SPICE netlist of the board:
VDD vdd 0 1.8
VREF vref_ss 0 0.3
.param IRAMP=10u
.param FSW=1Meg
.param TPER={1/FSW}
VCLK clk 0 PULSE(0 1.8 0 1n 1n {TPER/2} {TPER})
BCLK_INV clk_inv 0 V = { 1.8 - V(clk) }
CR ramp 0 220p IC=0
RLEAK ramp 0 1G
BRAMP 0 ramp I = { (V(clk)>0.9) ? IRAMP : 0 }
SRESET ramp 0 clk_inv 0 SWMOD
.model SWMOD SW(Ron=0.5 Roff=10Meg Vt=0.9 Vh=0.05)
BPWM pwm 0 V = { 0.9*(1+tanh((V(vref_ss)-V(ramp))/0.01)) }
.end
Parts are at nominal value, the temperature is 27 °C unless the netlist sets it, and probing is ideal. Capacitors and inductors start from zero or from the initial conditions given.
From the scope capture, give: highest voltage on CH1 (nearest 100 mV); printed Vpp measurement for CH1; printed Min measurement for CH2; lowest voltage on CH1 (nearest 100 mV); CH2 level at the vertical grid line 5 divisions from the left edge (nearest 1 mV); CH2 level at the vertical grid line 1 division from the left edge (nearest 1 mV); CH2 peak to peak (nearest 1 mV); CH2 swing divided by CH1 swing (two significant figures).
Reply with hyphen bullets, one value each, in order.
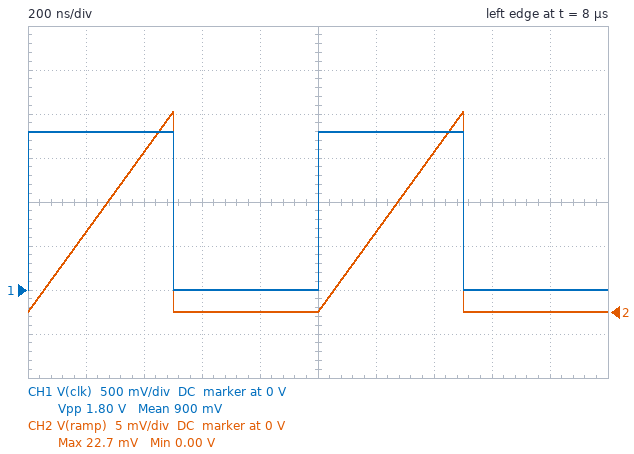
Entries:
- 1.8 V
- 1.80 V
- 0.00 V
- 0 V
- 0 V
- 9 mV
- 23 mV
- 0.013
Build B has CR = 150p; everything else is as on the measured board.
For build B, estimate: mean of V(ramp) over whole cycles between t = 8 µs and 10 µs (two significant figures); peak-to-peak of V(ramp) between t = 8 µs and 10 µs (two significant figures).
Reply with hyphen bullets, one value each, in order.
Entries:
- 8.4 mV
- 33 mV
